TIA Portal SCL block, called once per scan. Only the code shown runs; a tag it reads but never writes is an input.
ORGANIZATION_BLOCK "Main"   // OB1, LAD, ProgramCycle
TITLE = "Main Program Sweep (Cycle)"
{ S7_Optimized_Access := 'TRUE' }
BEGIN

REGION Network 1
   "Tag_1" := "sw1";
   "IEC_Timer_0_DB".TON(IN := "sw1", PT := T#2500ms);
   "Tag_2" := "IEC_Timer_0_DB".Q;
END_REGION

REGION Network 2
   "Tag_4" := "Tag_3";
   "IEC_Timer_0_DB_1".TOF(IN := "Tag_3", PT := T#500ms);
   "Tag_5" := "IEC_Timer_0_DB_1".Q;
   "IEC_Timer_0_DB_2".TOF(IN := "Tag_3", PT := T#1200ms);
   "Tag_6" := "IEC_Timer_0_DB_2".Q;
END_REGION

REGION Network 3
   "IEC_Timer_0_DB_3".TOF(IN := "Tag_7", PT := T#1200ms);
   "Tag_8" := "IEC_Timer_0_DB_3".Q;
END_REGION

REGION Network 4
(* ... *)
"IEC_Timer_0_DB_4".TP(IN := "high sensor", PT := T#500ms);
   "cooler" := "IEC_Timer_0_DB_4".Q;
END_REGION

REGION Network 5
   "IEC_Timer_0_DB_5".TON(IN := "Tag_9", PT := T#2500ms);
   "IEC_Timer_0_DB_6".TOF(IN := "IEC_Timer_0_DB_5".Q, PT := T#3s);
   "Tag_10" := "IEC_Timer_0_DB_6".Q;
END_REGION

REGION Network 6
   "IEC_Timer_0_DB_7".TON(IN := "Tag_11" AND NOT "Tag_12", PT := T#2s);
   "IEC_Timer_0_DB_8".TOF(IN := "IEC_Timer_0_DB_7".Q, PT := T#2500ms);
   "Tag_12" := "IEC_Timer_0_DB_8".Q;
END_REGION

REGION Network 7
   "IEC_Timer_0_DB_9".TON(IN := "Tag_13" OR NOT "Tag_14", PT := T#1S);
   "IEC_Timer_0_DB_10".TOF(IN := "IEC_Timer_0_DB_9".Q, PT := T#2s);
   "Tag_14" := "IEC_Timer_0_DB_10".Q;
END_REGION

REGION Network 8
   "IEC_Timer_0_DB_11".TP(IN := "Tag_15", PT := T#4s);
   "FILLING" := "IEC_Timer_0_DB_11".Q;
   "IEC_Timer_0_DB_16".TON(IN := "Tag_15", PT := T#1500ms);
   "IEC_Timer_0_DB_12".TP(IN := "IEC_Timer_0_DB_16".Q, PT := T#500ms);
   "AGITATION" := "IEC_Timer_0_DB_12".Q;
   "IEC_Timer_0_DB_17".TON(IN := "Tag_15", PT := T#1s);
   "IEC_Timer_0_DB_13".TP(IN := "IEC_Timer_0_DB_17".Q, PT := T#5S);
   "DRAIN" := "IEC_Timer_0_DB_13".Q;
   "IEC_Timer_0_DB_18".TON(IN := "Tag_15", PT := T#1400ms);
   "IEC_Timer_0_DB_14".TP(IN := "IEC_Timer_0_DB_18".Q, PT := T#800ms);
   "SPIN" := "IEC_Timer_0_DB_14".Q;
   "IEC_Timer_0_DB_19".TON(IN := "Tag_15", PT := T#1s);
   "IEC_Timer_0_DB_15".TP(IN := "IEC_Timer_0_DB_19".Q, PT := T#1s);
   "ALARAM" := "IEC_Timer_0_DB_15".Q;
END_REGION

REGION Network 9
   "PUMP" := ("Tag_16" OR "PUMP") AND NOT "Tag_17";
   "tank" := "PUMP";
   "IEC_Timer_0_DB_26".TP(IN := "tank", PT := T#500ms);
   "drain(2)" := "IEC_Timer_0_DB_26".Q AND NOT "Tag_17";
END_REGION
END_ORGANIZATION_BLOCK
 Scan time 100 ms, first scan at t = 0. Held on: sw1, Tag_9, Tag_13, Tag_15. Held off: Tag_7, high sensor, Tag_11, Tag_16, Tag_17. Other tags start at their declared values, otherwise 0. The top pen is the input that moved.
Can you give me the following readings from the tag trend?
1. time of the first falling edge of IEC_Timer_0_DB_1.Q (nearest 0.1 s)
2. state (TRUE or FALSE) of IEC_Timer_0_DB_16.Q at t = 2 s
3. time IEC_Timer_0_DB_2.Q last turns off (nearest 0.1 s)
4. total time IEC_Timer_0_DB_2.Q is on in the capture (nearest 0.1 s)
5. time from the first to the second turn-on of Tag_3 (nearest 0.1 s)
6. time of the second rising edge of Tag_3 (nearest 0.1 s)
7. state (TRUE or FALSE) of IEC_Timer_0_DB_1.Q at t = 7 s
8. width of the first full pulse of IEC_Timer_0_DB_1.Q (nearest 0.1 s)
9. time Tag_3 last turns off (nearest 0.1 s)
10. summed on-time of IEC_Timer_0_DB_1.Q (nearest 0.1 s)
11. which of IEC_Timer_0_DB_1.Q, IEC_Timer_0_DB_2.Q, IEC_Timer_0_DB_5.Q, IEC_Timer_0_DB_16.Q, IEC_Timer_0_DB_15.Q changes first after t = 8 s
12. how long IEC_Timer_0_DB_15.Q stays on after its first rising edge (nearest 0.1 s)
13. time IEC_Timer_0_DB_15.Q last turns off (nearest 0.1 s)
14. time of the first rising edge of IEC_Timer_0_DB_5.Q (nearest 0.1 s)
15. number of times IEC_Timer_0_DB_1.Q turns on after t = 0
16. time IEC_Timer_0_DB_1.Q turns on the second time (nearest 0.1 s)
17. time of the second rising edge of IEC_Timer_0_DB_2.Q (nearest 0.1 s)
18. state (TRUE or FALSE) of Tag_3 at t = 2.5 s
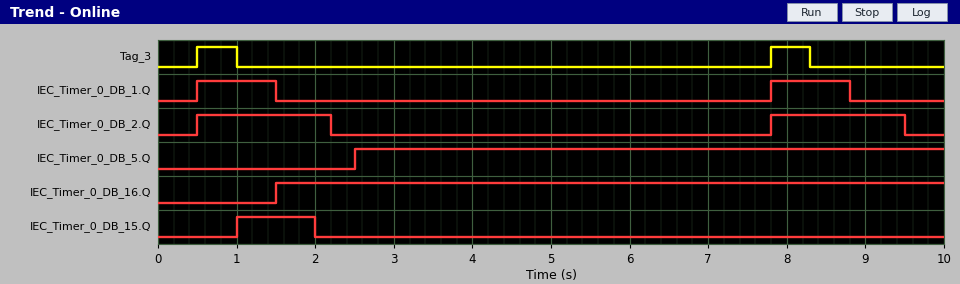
1.5 s
TRUE
9.5 s
3.4 s
7.3 s
7.8 s
FALSE
1.0 s
8.3 s
2.0 s
IEC_Timer_0_DB_1.Q
1.0 s
2.0 s
2.5 s
2
7.8 s
7.8 s
FALSE
